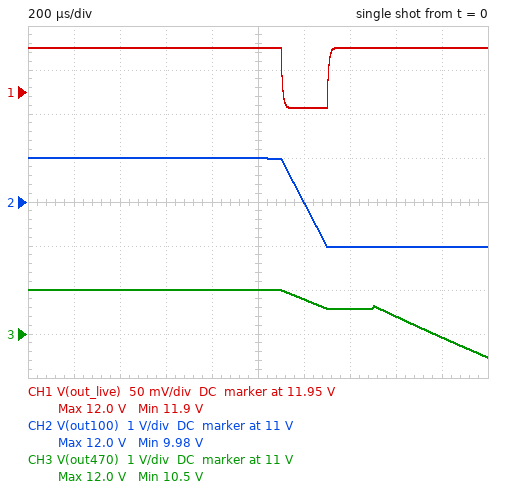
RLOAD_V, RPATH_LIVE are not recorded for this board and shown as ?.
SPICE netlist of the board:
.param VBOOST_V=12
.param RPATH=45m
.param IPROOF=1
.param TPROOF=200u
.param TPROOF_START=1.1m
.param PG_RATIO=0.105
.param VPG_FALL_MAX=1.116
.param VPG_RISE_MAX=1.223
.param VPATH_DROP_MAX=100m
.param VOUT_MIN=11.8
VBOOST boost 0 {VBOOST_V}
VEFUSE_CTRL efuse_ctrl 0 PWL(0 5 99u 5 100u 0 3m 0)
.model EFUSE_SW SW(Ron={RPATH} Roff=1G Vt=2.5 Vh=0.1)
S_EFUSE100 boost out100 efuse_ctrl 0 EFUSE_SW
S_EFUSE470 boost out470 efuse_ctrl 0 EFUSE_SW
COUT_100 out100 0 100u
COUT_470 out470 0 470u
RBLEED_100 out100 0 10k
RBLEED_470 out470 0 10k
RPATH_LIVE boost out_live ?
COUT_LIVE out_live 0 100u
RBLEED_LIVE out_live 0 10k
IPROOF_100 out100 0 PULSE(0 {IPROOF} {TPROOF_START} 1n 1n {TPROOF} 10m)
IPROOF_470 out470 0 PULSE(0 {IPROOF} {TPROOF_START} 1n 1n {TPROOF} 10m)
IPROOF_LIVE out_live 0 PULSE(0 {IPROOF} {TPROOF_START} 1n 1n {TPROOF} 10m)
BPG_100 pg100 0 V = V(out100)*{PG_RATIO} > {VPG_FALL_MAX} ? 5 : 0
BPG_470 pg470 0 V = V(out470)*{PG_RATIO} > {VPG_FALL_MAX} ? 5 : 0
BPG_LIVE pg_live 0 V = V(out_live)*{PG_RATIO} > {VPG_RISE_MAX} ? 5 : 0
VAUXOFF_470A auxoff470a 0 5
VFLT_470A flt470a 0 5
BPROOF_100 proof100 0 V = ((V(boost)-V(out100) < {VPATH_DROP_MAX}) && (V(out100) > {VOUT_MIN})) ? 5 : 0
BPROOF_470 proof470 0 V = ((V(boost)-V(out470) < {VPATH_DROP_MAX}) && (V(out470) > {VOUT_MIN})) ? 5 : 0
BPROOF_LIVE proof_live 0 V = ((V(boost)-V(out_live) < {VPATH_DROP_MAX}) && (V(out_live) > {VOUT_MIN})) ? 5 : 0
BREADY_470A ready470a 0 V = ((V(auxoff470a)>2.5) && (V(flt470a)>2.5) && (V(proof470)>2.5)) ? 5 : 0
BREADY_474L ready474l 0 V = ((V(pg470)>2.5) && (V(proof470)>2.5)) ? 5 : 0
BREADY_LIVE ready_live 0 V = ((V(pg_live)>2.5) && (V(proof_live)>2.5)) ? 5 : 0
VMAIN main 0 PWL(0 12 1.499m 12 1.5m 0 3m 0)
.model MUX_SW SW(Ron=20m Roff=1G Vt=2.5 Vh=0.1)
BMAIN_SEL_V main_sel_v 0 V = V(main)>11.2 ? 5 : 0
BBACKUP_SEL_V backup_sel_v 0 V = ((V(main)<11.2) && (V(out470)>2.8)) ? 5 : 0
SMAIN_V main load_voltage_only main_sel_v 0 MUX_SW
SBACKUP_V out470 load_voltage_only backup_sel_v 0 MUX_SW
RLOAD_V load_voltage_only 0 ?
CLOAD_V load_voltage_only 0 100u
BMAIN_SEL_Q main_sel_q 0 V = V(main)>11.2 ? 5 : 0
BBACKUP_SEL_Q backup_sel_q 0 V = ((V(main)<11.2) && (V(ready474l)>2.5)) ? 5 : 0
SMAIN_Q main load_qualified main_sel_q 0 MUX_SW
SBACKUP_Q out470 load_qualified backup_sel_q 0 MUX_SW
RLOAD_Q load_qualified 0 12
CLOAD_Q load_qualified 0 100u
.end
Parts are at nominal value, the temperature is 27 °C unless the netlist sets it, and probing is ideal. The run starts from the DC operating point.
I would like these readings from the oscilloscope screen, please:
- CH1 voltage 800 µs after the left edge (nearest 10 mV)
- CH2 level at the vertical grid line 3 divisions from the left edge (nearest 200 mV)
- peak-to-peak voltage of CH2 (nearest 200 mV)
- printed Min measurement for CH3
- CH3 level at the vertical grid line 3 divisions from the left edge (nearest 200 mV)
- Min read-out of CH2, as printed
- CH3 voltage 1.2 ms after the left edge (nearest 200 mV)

12.00 V
12.0 V
2.0 V
10.5 V
12.0 V
9.98 V
11.8 V
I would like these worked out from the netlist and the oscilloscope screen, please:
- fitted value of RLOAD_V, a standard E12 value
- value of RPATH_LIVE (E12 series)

8.2 Ω
0.068 Ω
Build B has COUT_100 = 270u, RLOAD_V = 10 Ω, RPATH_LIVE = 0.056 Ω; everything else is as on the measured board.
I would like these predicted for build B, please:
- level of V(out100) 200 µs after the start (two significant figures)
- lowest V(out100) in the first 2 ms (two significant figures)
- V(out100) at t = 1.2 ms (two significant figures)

12 V
11 V
12 V
